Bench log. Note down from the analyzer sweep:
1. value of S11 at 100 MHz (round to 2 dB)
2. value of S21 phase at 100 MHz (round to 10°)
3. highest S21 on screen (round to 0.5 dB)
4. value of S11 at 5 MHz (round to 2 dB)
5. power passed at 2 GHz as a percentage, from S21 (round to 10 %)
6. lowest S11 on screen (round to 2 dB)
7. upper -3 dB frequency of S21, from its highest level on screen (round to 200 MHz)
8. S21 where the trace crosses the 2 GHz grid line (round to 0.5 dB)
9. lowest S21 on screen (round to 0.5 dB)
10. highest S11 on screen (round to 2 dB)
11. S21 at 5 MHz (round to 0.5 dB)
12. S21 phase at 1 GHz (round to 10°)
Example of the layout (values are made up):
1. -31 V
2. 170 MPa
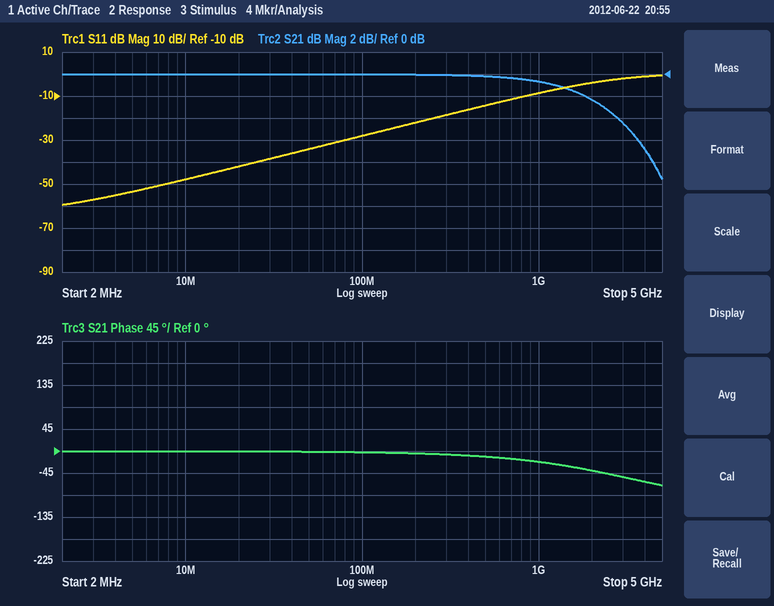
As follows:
1. -28 dB
2. 0°
3. 0.0 dB
4. -54 dB
5. 60 %
6. -60 dB
7. 2.4 GHz
8. -2.5 dB
9. -9.5 dB
10. 0 dB
11. 0.0 dB
12. -20°
